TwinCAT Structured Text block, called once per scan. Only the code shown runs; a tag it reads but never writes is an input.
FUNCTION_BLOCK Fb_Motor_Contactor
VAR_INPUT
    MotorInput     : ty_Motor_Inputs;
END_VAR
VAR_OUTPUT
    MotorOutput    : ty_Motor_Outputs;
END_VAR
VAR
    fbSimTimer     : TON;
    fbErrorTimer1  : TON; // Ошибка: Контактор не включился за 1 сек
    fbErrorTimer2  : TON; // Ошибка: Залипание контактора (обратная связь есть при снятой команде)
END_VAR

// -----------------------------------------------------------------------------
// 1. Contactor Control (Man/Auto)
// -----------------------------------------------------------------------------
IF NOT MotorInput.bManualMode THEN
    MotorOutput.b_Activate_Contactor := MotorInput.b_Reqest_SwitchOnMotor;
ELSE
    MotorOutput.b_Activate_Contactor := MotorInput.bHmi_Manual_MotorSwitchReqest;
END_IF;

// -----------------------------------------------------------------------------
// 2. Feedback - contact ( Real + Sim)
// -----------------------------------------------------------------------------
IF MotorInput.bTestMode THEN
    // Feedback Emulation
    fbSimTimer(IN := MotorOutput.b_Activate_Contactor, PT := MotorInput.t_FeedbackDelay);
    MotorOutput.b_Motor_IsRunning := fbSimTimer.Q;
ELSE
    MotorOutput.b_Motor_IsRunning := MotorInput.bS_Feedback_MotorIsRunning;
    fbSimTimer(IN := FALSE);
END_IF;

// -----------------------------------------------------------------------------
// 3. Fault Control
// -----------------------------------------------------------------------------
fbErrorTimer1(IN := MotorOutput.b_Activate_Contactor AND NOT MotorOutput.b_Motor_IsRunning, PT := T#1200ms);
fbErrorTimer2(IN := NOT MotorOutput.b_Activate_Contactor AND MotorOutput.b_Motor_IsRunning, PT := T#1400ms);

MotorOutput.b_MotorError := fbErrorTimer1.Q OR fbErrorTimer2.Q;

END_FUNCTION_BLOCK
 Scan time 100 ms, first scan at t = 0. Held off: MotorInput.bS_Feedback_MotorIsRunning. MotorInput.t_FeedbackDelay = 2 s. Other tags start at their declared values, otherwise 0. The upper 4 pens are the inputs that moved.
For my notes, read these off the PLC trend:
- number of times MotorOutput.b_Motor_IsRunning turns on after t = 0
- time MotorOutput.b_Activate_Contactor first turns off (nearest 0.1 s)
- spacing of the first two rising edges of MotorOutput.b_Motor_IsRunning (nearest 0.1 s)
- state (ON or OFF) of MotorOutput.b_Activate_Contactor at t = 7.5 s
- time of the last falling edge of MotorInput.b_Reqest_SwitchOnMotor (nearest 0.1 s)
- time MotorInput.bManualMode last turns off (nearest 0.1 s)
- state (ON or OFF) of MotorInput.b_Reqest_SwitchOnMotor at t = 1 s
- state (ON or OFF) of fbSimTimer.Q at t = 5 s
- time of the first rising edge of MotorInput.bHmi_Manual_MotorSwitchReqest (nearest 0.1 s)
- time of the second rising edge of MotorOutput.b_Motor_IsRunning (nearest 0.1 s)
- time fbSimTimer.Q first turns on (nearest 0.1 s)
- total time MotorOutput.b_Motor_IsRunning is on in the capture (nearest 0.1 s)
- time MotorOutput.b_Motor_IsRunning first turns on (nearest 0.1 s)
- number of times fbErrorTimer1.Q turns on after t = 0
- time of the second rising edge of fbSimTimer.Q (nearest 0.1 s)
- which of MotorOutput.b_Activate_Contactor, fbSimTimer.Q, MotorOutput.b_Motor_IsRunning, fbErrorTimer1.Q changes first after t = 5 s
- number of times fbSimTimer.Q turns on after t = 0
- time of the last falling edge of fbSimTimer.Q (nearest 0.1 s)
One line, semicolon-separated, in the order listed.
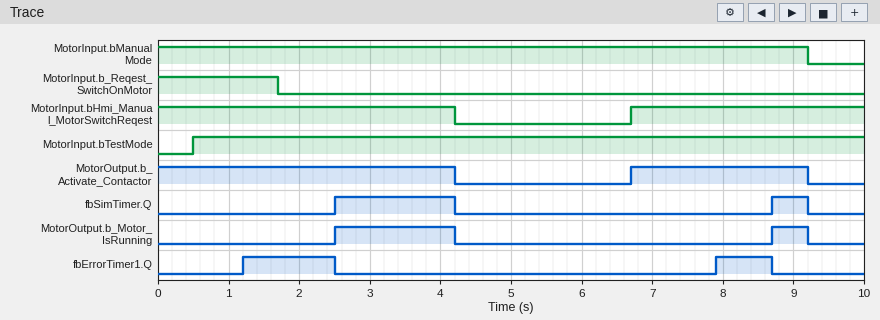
2; 4.2 s; 6.2 s; ON; 1.7 s; 9.2 s; ON; OFF; 6.7 s; 8.7 s; 2.5 s; 2.2 s; 2.5 s; 2; 8.7 s; MotorOutput.b_Activate_Contactor; 2; 9.2 s
